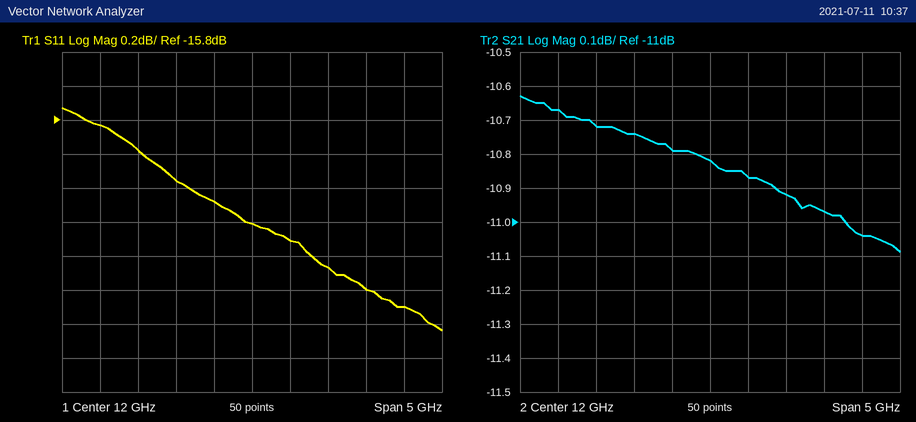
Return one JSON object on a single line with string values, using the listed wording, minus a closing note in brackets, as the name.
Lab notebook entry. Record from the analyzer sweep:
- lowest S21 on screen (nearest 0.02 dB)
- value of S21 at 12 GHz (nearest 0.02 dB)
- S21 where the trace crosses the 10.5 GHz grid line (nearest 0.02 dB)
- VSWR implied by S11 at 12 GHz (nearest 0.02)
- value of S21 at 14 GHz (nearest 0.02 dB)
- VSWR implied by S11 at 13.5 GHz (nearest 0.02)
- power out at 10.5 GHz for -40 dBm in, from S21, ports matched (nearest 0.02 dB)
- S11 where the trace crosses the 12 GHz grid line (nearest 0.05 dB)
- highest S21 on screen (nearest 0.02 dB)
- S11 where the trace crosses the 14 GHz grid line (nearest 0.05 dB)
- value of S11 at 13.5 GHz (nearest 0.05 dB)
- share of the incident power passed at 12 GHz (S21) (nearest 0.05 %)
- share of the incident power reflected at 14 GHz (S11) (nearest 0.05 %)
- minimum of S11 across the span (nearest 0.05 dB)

{"lowest S21 on screen": "-11.08 dB", "value of S21 at 12 GHz": "-10.82 dB", "S21 where the trace crosses the 10.5 GHz grid line": "-10.72 dB", "VSWR implied by S11 at 12 GHz": "1.36", "value of S21 at 14 GHz": "-11.04 dB", "VSWR implied by S11 at 13.5 GHz": "1.34", "power out at 10.5 GHz for -40 dBm in, from S21, ports matched": "-50.72 dBm", "S11 where the trace crosses the 12 GHz grid line": "-16.40 dB", "highest S21 on screen": "-10.62 dB", "S11 where the trace crosses the 14 GHz grid line": "-16.90 dB", "value of S11 at 13.5 GHz": "-16.80 dB", "share of the incident power passed at 12 GHz (S21)": "8.30 %", "share of the incident power reflected at 14 GHz (S11)": "2.05 %", "minimum of S11 across the span": "-17.05 dB"}
